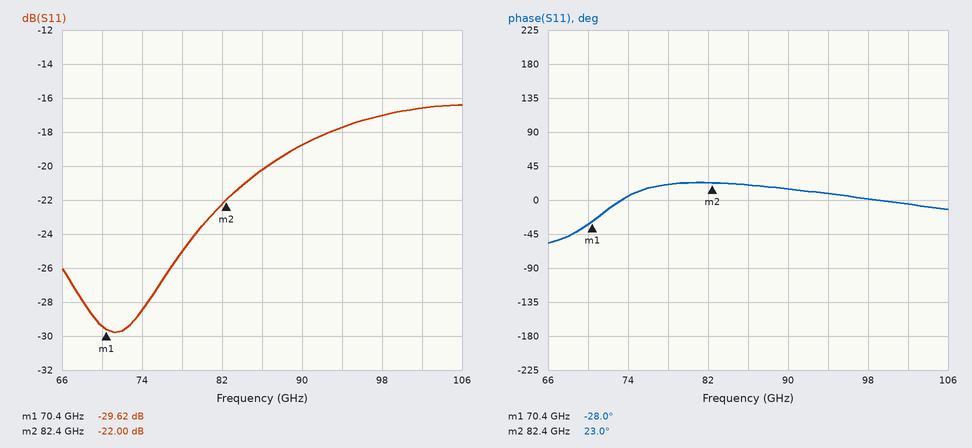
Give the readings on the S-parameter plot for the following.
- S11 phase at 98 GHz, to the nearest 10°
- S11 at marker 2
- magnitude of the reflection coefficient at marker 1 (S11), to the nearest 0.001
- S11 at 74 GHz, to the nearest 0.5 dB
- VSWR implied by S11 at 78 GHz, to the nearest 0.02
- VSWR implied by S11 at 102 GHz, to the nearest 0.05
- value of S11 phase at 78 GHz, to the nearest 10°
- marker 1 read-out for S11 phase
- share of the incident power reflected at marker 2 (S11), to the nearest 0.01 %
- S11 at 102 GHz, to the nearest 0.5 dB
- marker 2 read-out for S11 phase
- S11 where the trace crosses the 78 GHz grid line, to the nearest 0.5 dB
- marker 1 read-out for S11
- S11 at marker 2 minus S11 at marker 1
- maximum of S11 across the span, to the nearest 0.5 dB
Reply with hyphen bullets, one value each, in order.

- 0°
- -22.00 dB
- 0.033
- -28.5 dB
- 1.12
- 1.35
- 20°
- -28.0°
- 0.63 %
- -16.5 dB
- 23.0°
- -25.0 dB
- -29.62 dB
- 7.62 dB
- -16.5 dB
